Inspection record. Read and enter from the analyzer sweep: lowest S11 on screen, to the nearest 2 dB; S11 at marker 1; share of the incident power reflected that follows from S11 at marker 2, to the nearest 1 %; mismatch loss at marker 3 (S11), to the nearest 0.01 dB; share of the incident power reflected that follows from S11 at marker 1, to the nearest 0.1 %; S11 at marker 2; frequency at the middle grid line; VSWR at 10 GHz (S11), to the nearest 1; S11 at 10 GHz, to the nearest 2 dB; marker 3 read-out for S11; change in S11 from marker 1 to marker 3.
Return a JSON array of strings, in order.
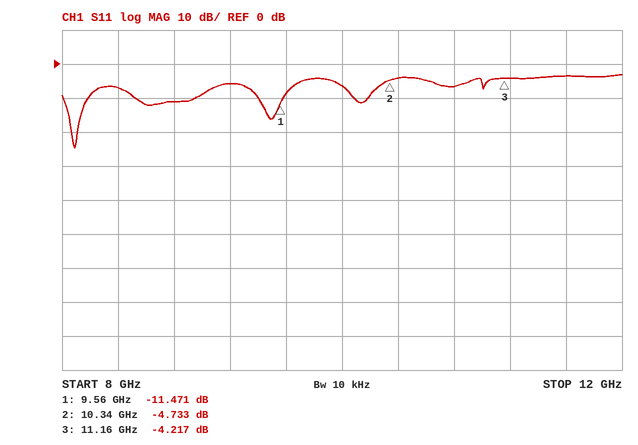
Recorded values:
["-24 dB", "-11.471 dB", "34 %", "2.07 dB", "7.1 %", "-4.733 dB", "10 GHz", "3", "-6 dB", "-4.217 dB", "7.254 dB"]
